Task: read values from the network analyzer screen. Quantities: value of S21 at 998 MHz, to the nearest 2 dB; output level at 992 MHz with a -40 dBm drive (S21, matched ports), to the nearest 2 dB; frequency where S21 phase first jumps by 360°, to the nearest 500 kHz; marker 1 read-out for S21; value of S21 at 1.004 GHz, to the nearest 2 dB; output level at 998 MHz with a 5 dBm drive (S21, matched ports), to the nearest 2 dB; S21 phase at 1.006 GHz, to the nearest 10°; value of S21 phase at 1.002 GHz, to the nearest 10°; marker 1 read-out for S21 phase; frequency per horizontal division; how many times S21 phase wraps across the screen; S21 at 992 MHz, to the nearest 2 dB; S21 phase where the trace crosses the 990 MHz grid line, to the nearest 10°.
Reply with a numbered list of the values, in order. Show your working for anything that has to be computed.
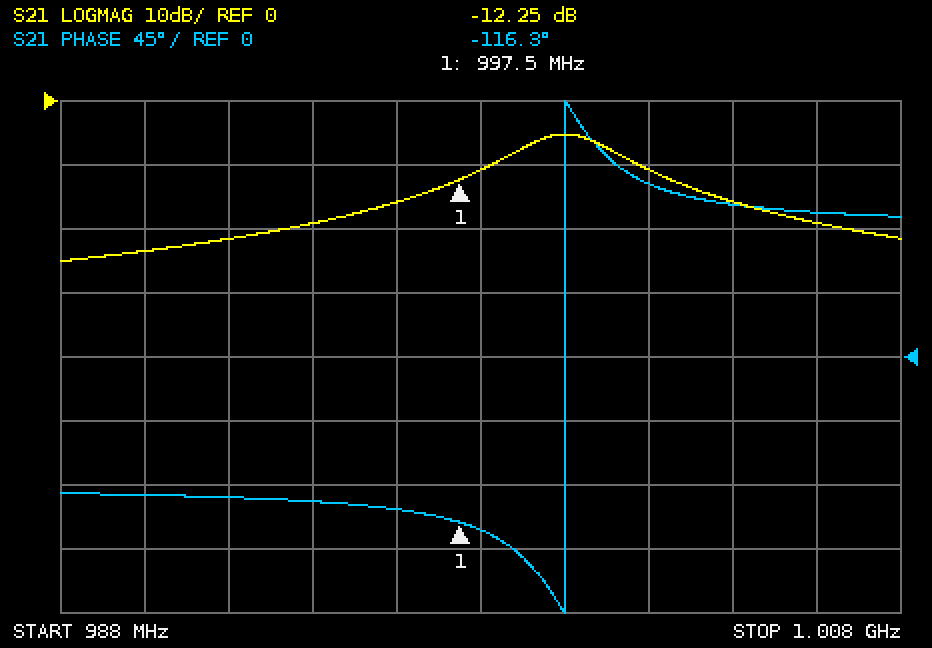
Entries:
1. -10 dB
2. -40 dBm + (-22 dB) = -62 dBm
3. 1.0000 GHz
4. -12.25 dB
5. -16 dB
6. 5 dBm + (-10 dB) = -6 dBm
7. 100°
8. 120°
9. -116.3°
10. 2 MHz
11. 1
12. -22 dB
13. -100°
